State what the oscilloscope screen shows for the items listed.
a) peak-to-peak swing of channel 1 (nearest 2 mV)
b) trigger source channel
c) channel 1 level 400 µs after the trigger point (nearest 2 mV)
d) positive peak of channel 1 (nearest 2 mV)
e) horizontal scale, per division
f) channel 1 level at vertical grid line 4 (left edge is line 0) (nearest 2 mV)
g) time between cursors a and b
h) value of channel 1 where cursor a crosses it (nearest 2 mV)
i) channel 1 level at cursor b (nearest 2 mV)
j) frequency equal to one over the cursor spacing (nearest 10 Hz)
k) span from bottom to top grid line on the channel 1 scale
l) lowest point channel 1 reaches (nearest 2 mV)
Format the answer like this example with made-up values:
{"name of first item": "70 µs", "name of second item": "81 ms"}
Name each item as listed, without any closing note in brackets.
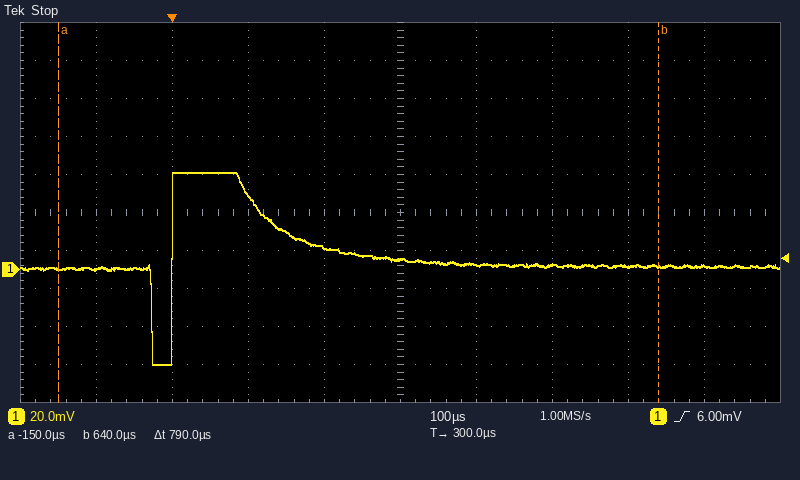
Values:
{"peak-to-peak swing of channel 1": "102 mV", "trigger source channel": "channel 1", "channel 1 level 400 µs after the trigger point": "2 mV", "positive peak of channel 1": "52 mV", "horizontal scale, per division": "100 µs", "channel 1 level at vertical grid line 4 (left edge is line 0)": "12 mV", "time between cursors a and b": "790 µs", "value of channel 1 where cursor a crosses it": "0 mV", "channel 1 level at cursor b": "2 mV", "frequency equal to one over the cursor spacing": "1.27 kHz", "span from bottom to top grid line on the channel 1 scale": "200 mV", "lowest point channel 1 reaches": "-50 mV"}
